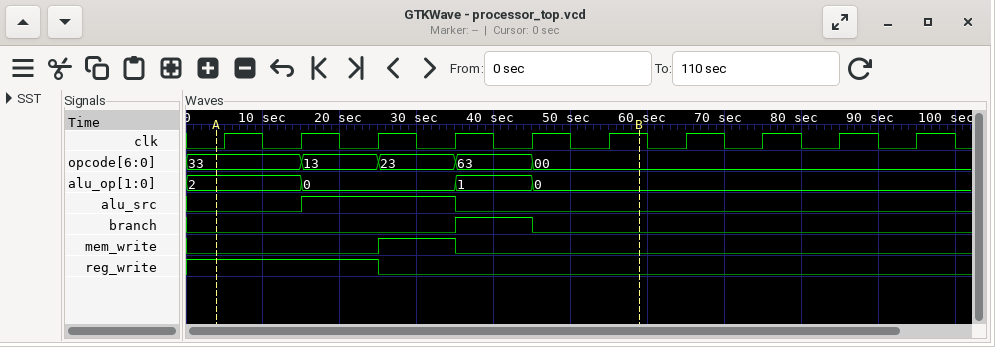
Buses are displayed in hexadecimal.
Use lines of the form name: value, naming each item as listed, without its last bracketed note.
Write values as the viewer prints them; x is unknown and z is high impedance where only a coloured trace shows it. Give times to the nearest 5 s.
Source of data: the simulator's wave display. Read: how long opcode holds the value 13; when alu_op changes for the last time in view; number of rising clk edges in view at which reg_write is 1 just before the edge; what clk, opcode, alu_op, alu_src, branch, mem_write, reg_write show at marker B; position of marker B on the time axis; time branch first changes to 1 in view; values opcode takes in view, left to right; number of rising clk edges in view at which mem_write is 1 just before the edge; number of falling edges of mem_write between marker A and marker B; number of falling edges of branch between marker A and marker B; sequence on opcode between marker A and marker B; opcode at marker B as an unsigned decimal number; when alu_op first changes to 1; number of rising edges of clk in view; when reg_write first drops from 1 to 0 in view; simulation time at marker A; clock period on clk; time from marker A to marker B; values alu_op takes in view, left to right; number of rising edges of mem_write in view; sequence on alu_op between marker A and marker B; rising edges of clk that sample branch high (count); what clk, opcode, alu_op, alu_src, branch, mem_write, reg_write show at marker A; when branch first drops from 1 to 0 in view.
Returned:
how long opcode holds the value 13: 10 s
when alu_op changes for the last time in view: 45 s
number of rising clk edges in view at which reg_write is 1 just before the edge: 3
what clk, opcode, alu_op, alu_src, branch, mem_write, reg_write show at marker B: clk=1, opcode=00, alu_op=0, alu_src=0, branch=0, mem_write=0, reg_write=0
position of marker B on the time axis: 60 s
time branch first changes to 1 in view: 35 s
values opcode takes in view, left to right: 33, 13, 23, 63, 00
number of rising clk edges in view at which mem_write is 1 just before the edge: 1
number of falling edges of mem_write between marker A and marker B: 1
number of falling edges of branch between marker A and marker B: 1
sequence on opcode between marker A and marker B: 33, 13, 23, 63, 00
opcode at marker B as an unsigned decimal number: 0
when alu_op first changes to 1: 35 s
number of rising edges of clk in view: 10
when reg_write first drops from 1 to 0 in view: 25 s
simulation time at marker A: 5 s
clock period on clk: 10 s
time from marker A to marker B: 55 s
values alu_op takes in view, left to right: 2, 0, 1, 0
number of rising edges of mem_write in view: 1
sequence on alu_op between marker A and marker B: 2, 0, 1, 0
rising edges of clk that sample branch high: 1
what clk, opcode, alu_op, alu_src, branch, mem_write, reg_write show at marker A: clk=0, opcode=33, alu_op=2, alu_src=0, branch=0, mem_write=0, reg_write=1
when branch first drops from 1 to 0 in view: 45 s
